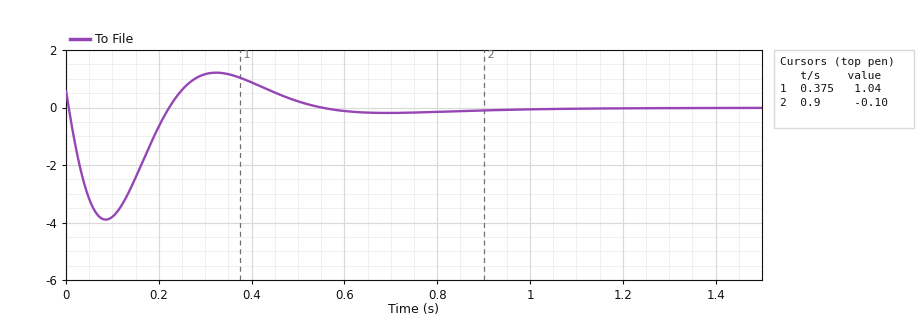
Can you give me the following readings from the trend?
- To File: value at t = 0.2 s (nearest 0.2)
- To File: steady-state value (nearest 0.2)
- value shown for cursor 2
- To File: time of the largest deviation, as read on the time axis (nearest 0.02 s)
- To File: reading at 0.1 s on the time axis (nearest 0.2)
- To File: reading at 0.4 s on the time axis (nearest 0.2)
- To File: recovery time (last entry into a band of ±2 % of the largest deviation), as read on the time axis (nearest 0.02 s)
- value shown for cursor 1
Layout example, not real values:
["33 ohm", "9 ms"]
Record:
["-0.6", "0.0", "-0.10", "0.08 s", "-3.8", "0.8", "0.92 s", "1.04"]
